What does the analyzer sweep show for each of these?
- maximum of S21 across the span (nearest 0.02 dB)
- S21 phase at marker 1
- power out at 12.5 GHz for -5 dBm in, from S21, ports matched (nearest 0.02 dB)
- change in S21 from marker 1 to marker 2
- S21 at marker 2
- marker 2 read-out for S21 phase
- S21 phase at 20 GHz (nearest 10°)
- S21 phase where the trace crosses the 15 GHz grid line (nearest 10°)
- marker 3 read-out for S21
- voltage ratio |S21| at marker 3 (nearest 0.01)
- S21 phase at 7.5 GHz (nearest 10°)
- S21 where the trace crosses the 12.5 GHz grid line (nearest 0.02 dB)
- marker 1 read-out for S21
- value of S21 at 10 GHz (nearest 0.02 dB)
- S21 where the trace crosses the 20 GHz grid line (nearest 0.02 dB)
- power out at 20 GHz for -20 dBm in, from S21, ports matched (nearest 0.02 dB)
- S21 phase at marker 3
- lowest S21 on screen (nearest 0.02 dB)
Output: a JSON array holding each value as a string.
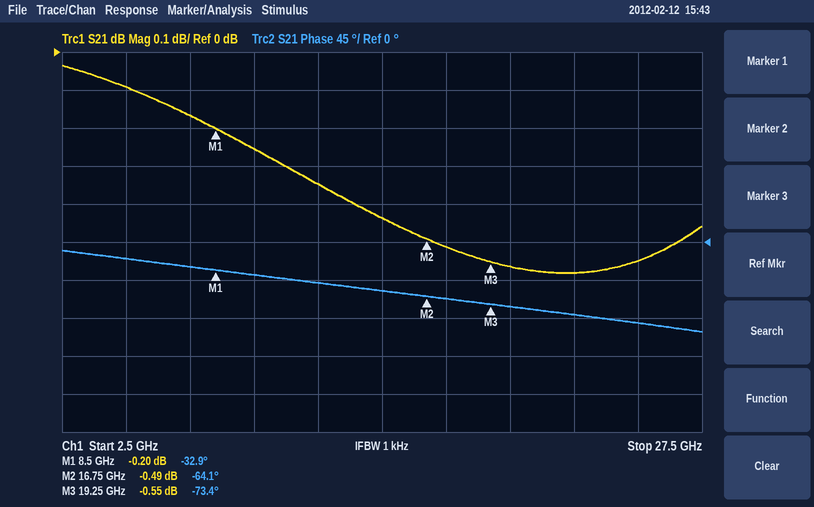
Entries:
["-0.04 dB", "-32.9°", "-5.34 dBm", "-0.29 dB", "-0.49 dB", "-64.1°", "-80°", "-60°", "-0.55 dB", "0.94", "-30°", "-0.34 dB", "-0.20 dB", "-0.26 dB", "-0.56 dB", "-20.56 dBm", "-73.4°", "-0.58 dB"]
